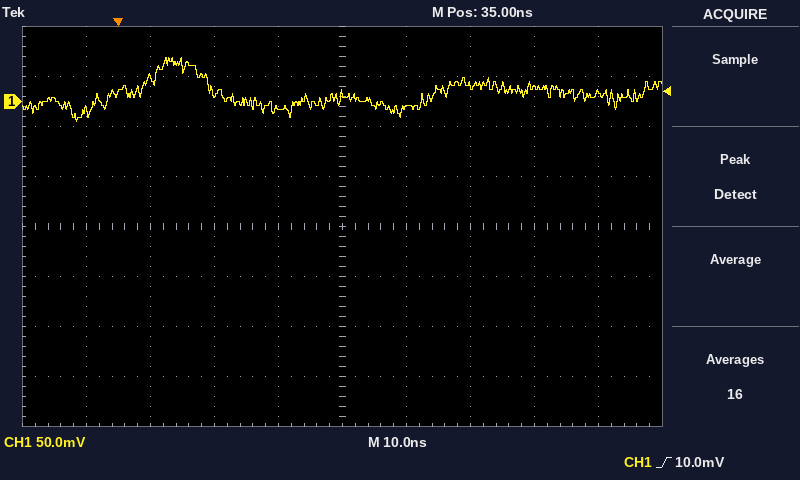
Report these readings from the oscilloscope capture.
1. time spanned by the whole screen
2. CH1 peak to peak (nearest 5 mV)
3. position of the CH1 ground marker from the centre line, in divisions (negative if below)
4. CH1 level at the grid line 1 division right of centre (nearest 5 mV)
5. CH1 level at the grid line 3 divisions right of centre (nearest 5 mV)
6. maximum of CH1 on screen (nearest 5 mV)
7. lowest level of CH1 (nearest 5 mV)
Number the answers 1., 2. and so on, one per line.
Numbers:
1. 100 ns
2. 65 mV
3. +2.5 div
4. -5 mV
5. 15 mV
6. 45 mV
7. -20 mV
